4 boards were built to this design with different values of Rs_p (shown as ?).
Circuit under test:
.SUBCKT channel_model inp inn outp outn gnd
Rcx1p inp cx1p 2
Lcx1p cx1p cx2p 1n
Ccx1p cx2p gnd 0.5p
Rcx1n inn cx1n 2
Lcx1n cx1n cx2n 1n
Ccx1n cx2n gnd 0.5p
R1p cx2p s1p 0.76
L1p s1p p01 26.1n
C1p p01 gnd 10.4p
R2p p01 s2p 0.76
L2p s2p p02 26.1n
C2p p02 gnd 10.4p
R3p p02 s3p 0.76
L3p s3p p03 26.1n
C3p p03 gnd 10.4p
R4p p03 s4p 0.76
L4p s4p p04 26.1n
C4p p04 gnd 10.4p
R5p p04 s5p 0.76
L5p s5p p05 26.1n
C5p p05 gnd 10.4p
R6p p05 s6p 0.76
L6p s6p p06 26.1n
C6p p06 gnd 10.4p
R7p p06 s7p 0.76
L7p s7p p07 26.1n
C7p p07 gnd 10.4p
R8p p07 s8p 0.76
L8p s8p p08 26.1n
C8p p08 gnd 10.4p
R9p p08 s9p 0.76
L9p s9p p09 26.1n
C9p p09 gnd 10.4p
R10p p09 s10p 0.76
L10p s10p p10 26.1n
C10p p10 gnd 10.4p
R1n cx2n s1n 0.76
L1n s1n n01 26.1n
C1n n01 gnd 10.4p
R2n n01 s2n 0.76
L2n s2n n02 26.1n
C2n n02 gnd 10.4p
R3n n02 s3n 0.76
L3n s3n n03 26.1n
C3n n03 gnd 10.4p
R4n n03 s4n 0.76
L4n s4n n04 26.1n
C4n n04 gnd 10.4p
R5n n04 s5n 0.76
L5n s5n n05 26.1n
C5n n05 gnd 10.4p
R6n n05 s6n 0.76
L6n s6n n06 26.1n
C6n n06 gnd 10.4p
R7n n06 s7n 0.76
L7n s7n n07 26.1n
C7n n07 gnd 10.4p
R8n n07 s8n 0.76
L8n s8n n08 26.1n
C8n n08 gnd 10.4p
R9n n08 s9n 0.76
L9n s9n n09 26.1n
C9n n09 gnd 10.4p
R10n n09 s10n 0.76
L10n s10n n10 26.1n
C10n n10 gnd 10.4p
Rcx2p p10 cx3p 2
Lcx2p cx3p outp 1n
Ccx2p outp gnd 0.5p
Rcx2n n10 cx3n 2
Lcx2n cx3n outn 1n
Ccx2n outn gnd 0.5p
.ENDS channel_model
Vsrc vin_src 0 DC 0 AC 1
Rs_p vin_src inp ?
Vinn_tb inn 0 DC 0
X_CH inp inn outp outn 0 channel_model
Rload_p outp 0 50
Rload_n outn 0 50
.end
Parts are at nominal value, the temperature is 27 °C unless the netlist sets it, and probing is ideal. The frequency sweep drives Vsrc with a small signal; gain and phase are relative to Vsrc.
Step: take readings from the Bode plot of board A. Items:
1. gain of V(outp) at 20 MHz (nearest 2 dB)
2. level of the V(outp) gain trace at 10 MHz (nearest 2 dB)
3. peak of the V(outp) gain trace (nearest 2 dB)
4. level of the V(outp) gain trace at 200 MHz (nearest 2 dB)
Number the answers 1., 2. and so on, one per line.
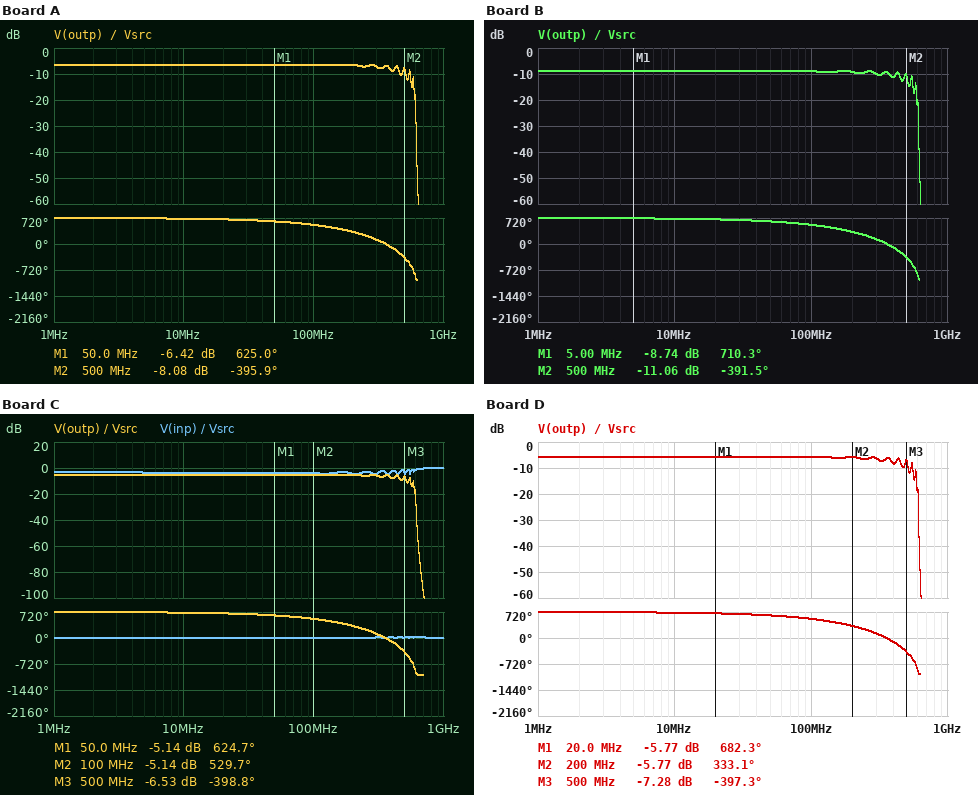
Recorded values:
1. -6 dB
2. -6 dB
3. -6 dB
4. -6 dB
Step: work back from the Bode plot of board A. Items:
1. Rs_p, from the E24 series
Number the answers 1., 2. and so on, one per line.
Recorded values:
1. 43 Ω
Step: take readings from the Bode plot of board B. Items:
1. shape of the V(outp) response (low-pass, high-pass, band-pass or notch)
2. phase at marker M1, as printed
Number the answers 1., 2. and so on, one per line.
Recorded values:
1. low-pass
2. 710.3 deg
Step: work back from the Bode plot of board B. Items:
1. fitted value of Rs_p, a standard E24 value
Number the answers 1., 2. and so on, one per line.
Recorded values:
1. 75 Ω
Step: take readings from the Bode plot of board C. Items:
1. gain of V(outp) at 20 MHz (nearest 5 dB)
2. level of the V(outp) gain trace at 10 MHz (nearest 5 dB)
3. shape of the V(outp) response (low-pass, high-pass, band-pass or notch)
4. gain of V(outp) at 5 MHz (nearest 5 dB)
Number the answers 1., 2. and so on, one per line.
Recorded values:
1. -5 dB
2. -5 dB
3. low-pass
4. -5 dB
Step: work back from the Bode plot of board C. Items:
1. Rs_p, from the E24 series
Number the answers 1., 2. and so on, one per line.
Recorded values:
1. 30 Ω
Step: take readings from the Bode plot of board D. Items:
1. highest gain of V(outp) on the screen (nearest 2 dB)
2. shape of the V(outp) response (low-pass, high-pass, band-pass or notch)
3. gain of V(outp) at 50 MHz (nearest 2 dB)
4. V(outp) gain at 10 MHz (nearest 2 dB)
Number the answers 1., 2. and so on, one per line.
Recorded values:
1. -6 dB
2. low-pass
3. -6 dB
4. -6 dB
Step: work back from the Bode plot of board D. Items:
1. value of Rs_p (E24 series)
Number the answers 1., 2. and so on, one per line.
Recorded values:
1. 36 Ω
